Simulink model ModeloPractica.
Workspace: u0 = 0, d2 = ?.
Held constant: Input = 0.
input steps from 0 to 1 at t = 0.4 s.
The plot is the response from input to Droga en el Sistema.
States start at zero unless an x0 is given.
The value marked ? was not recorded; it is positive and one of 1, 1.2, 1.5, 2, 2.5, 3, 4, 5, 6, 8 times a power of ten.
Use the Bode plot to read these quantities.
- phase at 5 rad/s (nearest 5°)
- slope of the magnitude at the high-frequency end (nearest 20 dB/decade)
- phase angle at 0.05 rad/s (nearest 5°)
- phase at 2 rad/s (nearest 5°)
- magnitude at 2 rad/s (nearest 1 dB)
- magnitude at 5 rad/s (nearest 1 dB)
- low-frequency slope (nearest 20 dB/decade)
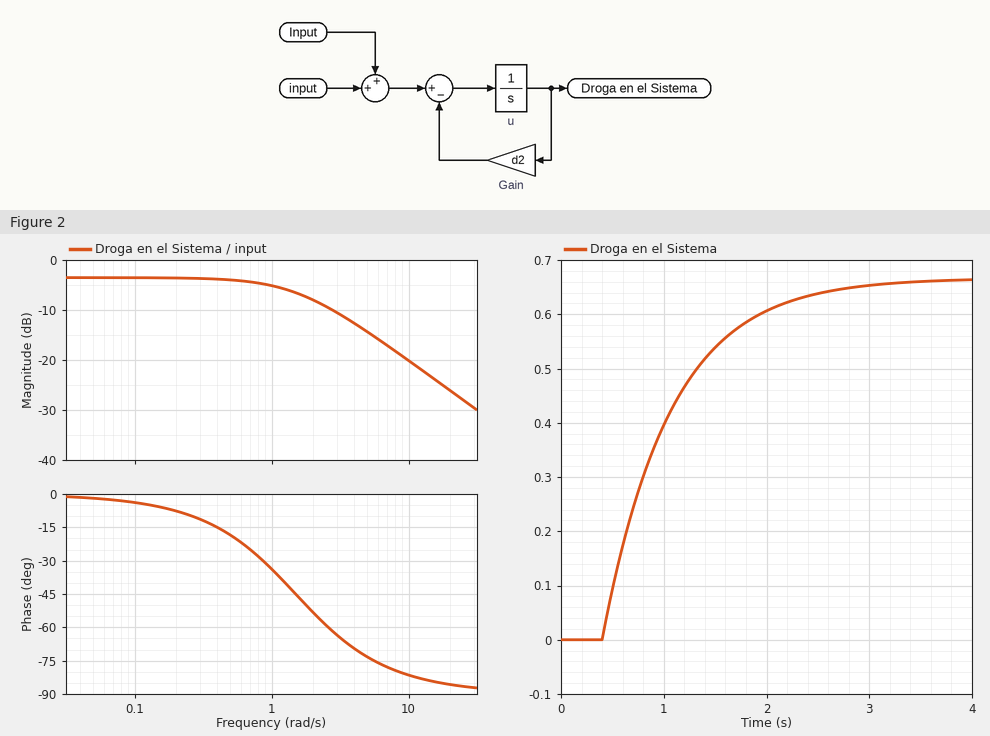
-75°
-20 dB/decade
0°
-55°
-8 dB
-14 dB
0 dB/decade
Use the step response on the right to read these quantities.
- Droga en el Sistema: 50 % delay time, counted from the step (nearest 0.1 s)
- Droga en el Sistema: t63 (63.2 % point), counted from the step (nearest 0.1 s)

0.5 s
0.7 s
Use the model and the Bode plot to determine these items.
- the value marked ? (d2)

1.5
